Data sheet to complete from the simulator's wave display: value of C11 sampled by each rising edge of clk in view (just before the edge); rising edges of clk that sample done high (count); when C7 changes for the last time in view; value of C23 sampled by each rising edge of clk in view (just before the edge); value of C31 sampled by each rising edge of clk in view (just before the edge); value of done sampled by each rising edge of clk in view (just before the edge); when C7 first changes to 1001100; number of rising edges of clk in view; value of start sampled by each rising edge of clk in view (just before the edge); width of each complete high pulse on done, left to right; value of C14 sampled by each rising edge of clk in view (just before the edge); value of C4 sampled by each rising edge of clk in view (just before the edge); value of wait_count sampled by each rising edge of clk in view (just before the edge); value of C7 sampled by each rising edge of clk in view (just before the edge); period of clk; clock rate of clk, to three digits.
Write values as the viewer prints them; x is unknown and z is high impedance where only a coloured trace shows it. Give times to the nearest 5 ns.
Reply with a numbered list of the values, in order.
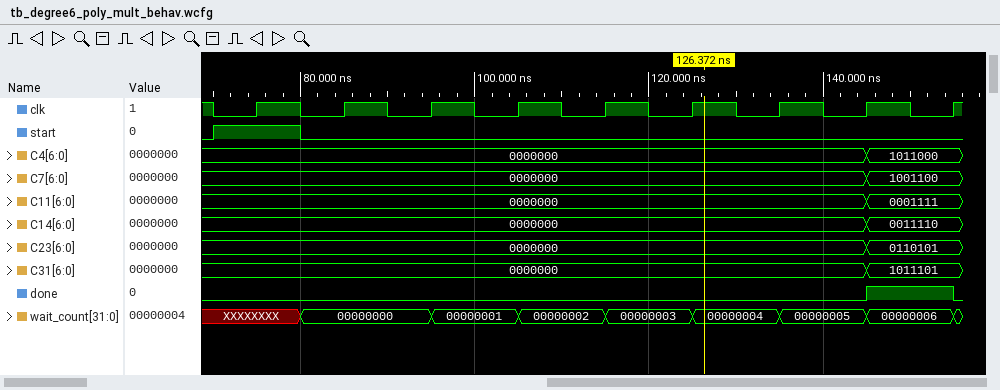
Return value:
1. 0000000, 0000000, 0000000, 0000000, 0000000, 0000000, 0000000, 0000000, 0001111
2. 1
3. 145 ns
4. 0000000, 0000000, 0000000, 0000000, 0000000, 0000000, 0000000, 0000000, 0110101
5. 0000000, 0000000, 0000000, 0000000, 0000000, 0000000, 0000000, 0000000, 1011101
6. 0 0 0 0 0 0 0 0 1
7. 145 ns
8. 9
9. 1 0 0 0 0 0 0 0 0
10. 10 ns
11. 0000000, 0000000, 0000000, 0000000, 0000000, 0000000, 0000000, 0000000, 0011110
12. 0000000, 0000000, 0000000, 0000000, 0000000, 0000000, 0000000, 0000000, 1011000
13. XXXXXXXX, 00000000, 00000000, 00000001, 00000002, 00000003, 00000004, 00000005, 00000006
14. 0000000, 0000000, 0000000, 0000000, 0000000, 0000000, 0000000, 0000000, 1001100
15. 10 ns
16. 100 MHz
